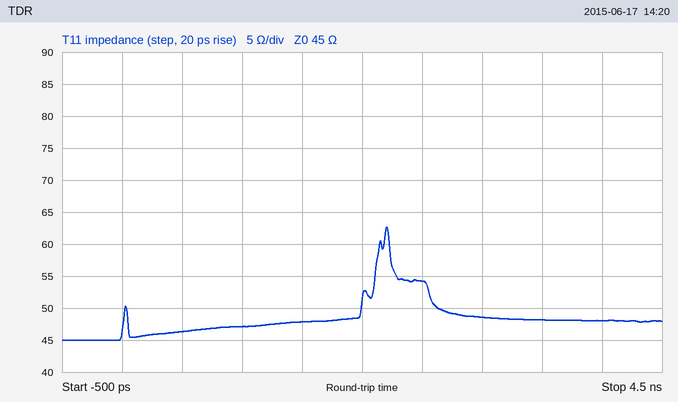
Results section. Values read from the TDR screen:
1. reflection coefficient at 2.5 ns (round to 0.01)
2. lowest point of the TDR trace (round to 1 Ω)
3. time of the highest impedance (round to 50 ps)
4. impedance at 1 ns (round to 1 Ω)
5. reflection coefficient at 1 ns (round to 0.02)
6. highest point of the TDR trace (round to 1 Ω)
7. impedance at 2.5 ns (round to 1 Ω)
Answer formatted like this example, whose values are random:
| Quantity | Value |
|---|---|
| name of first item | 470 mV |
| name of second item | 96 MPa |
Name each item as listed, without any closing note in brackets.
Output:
| Quantity | Value |
|---|---|
| reflection coefficient at 2.5 ns | +0.09 |
| lowest point of the TDR trace | 45 Ω |
| time of the highest impedance | 2.20 ns |
| impedance at 1 ns | 47 Ω |
| reflection coefficient at 1 ns | +0.02 |
| highest point of the TDR trace | 63 Ω |
| impedance at 2.5 ns | 54 Ω |
